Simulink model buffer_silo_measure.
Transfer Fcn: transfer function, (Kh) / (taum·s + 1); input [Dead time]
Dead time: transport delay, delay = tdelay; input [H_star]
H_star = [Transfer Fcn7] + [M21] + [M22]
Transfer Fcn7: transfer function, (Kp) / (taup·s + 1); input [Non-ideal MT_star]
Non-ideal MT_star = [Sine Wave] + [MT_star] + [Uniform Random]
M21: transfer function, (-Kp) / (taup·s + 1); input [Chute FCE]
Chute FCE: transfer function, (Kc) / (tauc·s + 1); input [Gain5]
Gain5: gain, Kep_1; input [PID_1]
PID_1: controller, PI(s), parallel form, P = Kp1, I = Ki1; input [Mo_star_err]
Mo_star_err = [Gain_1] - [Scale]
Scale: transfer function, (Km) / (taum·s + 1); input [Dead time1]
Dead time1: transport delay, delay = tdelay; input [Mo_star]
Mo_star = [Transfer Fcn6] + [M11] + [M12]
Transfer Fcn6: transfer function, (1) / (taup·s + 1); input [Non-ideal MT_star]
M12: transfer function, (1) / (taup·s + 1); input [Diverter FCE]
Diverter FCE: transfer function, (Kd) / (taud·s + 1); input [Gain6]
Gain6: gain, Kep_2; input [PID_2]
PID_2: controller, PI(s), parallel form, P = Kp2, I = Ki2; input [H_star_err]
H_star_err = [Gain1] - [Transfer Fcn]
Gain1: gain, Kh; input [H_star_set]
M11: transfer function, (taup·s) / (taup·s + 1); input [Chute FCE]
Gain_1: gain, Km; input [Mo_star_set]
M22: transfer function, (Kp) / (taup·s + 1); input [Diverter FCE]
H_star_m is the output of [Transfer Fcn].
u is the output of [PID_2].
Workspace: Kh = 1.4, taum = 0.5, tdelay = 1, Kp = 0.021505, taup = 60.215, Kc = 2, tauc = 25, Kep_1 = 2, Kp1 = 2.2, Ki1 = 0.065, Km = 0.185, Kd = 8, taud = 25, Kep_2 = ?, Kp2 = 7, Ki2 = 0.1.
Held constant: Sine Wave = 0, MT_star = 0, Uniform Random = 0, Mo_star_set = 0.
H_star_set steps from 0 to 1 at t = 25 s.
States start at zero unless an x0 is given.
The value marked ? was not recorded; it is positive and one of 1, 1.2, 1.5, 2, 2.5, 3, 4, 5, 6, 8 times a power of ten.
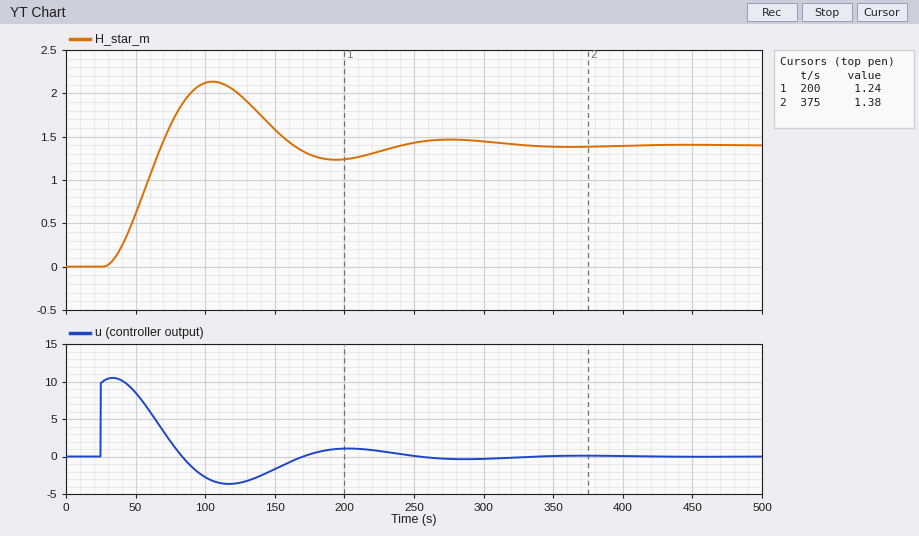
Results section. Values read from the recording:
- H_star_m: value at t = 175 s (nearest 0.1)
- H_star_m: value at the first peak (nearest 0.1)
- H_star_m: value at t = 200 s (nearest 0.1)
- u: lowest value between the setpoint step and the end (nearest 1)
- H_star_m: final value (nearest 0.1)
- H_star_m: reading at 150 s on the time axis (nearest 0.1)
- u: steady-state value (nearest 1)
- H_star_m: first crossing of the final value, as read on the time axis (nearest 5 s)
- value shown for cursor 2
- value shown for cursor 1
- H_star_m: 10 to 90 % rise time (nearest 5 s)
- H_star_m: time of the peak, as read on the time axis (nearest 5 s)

1.3
2.1
1.2
-4
1.4
1.6
0
70 s
1.38
1.24
30 s
105 s
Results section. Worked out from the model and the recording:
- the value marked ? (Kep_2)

2
